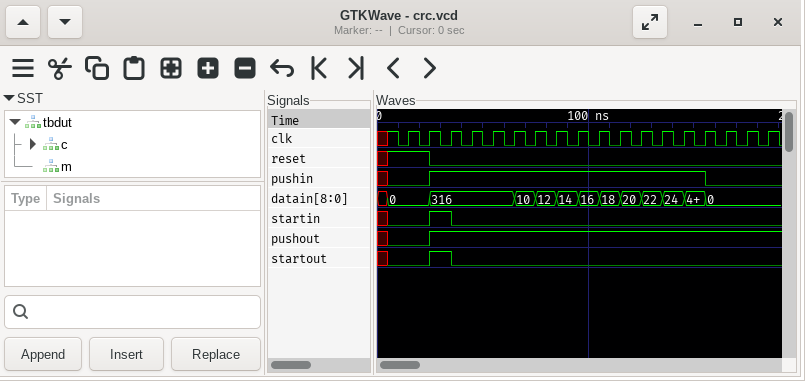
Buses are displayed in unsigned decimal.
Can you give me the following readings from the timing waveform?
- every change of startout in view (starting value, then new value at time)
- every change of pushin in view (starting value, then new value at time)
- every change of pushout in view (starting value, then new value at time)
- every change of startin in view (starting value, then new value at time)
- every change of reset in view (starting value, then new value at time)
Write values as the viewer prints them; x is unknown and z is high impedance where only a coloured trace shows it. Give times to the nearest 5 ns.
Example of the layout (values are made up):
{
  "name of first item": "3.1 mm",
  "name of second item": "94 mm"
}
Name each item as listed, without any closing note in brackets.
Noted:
{
  "every change of startout in view": "x, 0 at 5 ns, 1 at 25 ns, 0 at 35 ns",
  "every change of pushin in view": "x, 0 at 5 ns, 1 at 25 ns, 0 at 155 ns",
  "every change of pushout in view": "x, 0 at 5 ns, 1 at 25 ns",
  "every change of startin in view": "x, 0 at 5 ns, 1 at 25 ns, 0 at 35 ns",
  "every change of reset in view": "x, 1 at 5 ns, 0 at 25 ns"
}
